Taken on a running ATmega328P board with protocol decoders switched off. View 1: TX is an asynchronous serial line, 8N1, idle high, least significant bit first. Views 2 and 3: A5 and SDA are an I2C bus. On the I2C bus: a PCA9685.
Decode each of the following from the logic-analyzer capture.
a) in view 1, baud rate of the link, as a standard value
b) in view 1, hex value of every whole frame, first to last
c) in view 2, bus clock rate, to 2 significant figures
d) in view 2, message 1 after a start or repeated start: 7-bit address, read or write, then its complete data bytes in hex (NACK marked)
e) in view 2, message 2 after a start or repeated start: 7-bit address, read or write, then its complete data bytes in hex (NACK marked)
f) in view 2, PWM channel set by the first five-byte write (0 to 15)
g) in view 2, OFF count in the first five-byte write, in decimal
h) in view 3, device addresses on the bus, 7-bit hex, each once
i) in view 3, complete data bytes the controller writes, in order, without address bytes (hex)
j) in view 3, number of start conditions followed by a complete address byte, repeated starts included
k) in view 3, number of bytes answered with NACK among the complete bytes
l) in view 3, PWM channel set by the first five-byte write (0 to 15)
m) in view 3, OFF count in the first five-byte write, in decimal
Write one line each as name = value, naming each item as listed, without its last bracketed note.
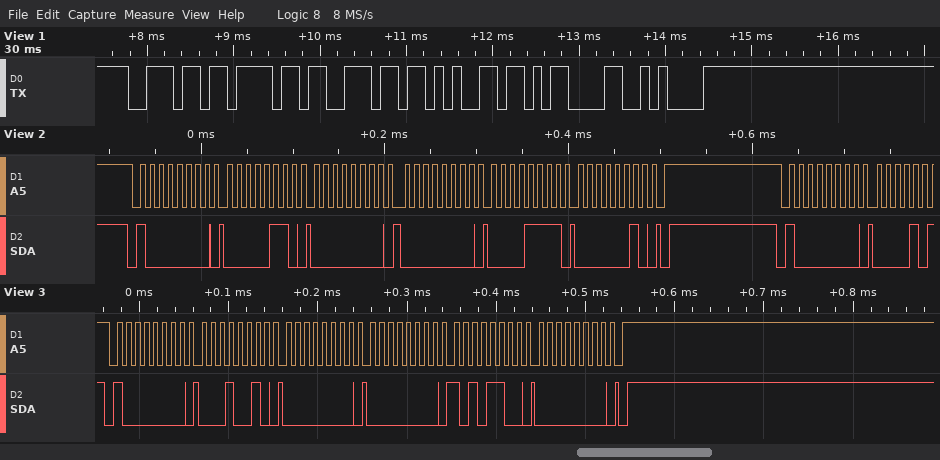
in view 1, baud rate of the link, as a standard value = 9600 baud
in view 1, hex value of every whole frame, first to last = 6E 6F 6E 65 0D 0A
in view 2, bus clock rate, to 2 significant figures = 100 kHz
in view 2, message 1 after a start or repeated start: 7-bit address, read or write, then its complete data bytes in hex = 0x40 write: 06 00 00 0F 02
in view 2, message 2 after a start or repeated start: 7-bit address, read or write, then its complete data bytes in hex = 0x40 write
in view 2, PWM channel set by the first five-byte write = 0
in view 2, OFF count in the first five-byte write, in decimal = 527
in view 3, device addresses on the bus, 7-bit hex, each once = 0x40
in view 3, complete data bytes the controller writes, in order, without address bytes = 12 00 00 AC 00
in view 3, number of start conditions followed by a complete address byte, repeated starts included = 1
in view 3, number of bytes answered with NACK among the complete bytes = 0
in view 3, PWM channel set by the first five-byte write = 3
in view 3, OFF count in the first five-byte write, in decimal = 172
